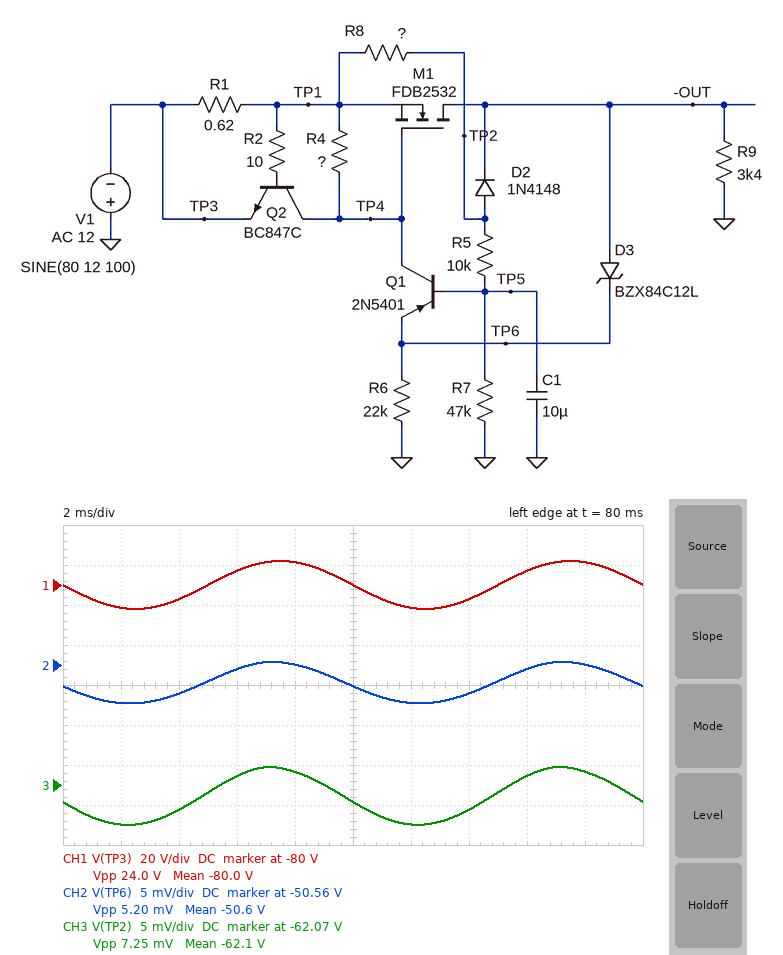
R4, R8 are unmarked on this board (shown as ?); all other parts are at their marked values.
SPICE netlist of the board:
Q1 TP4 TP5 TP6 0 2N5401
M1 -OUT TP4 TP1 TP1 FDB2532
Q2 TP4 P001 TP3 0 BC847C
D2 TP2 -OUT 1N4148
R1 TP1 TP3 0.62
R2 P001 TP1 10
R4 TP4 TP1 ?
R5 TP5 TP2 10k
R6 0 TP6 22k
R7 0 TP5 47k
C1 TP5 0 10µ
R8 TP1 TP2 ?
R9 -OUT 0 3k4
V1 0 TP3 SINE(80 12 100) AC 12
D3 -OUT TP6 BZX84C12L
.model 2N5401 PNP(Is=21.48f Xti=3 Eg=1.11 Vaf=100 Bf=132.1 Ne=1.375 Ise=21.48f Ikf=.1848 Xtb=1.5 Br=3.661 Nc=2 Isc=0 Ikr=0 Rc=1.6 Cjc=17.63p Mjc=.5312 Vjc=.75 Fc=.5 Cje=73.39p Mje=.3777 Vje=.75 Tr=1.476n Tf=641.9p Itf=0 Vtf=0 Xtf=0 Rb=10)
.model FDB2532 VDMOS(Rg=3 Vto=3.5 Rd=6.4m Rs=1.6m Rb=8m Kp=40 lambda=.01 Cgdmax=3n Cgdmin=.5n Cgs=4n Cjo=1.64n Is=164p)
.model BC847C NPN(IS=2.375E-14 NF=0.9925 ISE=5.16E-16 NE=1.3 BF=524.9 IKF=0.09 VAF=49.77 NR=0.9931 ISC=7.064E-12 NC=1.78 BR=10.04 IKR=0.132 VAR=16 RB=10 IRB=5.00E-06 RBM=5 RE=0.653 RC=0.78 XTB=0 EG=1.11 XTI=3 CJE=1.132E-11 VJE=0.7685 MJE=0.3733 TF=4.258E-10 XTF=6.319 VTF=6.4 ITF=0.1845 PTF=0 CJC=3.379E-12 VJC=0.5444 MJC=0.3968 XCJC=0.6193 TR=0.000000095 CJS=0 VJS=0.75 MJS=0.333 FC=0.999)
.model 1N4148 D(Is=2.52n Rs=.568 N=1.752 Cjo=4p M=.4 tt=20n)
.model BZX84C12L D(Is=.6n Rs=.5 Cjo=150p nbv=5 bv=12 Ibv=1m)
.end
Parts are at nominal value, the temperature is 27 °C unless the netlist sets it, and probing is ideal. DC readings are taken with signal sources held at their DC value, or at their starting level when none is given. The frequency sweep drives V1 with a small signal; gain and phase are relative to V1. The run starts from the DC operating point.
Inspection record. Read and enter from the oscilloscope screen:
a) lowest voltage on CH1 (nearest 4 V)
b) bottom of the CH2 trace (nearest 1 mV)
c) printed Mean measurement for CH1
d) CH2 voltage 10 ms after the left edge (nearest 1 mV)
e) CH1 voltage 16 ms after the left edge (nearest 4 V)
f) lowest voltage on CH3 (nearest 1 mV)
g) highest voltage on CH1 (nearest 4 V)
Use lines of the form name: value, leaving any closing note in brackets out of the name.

lowest voltage on CH1: -92 V
bottom of the CH2 trace: -50.570 V
printed Mean measurement for CH1: -80.0 V
CH2 voltage 10 ms after the left edge: -50.568 V
CH1 voltage 16 ms after the left edge: -72 V
lowest voltage on CH3: -62.075 V
highest voltage on CH1: -68 V
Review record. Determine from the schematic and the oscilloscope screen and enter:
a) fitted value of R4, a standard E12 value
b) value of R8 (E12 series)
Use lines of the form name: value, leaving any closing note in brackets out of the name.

fitted value of R4, a standard E12 value: 12 kΩ
value of R8: 560 kΩ
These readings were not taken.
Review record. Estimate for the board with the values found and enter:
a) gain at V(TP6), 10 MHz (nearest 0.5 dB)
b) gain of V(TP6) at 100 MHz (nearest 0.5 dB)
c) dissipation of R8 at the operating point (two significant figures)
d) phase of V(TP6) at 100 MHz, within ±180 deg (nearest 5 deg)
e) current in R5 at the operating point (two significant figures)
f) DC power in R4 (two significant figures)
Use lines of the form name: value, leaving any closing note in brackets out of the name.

gain at V(TP6), 10 MHz: -5.0 dB
gain of V(TP6) at 100 MHz: -10.0 dB
dissipation of R8 at the operating point: 570 µW
phase of V(TP6) at 100 MHz, within ±180 deg: -170 deg
current in R5 at the operating point: 1.1 mA
DC power in R4: 960 µW
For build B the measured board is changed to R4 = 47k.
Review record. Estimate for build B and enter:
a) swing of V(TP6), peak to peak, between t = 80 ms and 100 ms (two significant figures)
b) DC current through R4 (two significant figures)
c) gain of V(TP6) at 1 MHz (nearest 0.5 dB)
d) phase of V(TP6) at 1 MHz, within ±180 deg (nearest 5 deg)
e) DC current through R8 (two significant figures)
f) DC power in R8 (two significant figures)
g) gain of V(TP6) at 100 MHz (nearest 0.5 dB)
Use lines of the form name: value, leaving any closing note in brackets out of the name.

swing of V(TP6), peak to peak, between t = 80 ms and 100 ms: 6.2 mV
DC current through R4: 72 µA
gain of V(TP6) at 1 MHz: -2.5 dB
phase of V(TP6) at 1 MHz, within ±180 deg: -150 deg
DC current through R8: 31 µA
DC power in R8: 550 µW
gain of V(TP6) at 100 MHz: -9.5 dB
